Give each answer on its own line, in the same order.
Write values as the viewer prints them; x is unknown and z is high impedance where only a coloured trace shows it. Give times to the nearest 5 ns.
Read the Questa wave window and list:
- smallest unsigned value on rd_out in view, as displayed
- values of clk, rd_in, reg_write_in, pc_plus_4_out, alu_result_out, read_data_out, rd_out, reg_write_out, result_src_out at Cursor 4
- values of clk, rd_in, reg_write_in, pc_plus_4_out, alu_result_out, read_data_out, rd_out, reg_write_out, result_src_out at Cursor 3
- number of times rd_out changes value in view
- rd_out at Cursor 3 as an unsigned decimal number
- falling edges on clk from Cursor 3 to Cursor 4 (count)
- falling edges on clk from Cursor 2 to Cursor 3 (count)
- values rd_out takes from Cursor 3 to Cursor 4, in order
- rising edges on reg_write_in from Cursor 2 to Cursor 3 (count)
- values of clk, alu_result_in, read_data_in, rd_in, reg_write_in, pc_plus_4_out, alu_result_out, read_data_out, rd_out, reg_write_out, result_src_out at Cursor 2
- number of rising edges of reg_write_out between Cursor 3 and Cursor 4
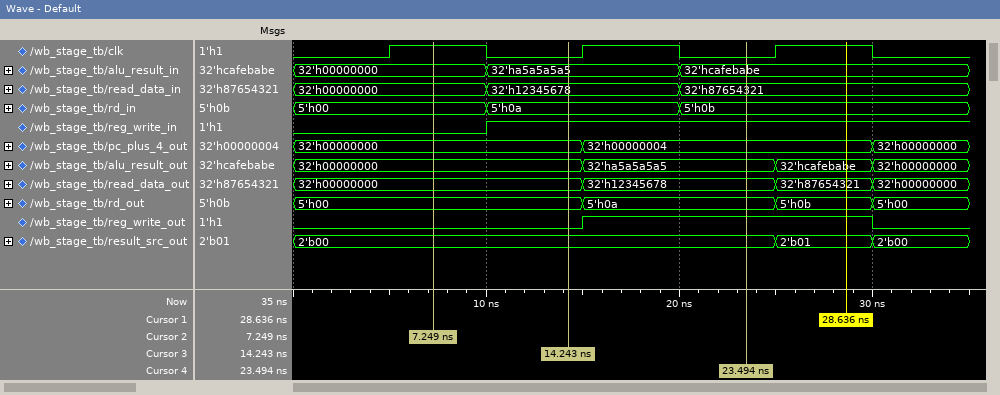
5'h00
clk=0, rd_in=5'h0b, reg_write_in=1, pc_plus_4_out=32'h00000004, alu_result_out=32'ha5a5a5a5, read_data_out=32'h12345678, rd_out=5'h0a, reg_write_out=1, result_src_out=2'b00
clk=0, rd_in=5'h0a, reg_write_in=1, pc_plus_4_out=32'h00000000, alu_result_out=32'h00000000, read_data_out=32'h00000000, rd_out=5'h00, reg_write_out=0, result_src_out=2'b00
3
0
1
1
5'h00, 5'h0a
1
clk=1, alu_result_in=32'h00000000, read_data_in=32'h00000000, rd_in=5'h00, reg_write_in=0, pc_plus_4_out=32'h00000000, alu_result_out=32'h00000000, read_data_out=32'h00000000, rd_out=5'h00, reg_write_out=0, result_src_out=2'b00
1
